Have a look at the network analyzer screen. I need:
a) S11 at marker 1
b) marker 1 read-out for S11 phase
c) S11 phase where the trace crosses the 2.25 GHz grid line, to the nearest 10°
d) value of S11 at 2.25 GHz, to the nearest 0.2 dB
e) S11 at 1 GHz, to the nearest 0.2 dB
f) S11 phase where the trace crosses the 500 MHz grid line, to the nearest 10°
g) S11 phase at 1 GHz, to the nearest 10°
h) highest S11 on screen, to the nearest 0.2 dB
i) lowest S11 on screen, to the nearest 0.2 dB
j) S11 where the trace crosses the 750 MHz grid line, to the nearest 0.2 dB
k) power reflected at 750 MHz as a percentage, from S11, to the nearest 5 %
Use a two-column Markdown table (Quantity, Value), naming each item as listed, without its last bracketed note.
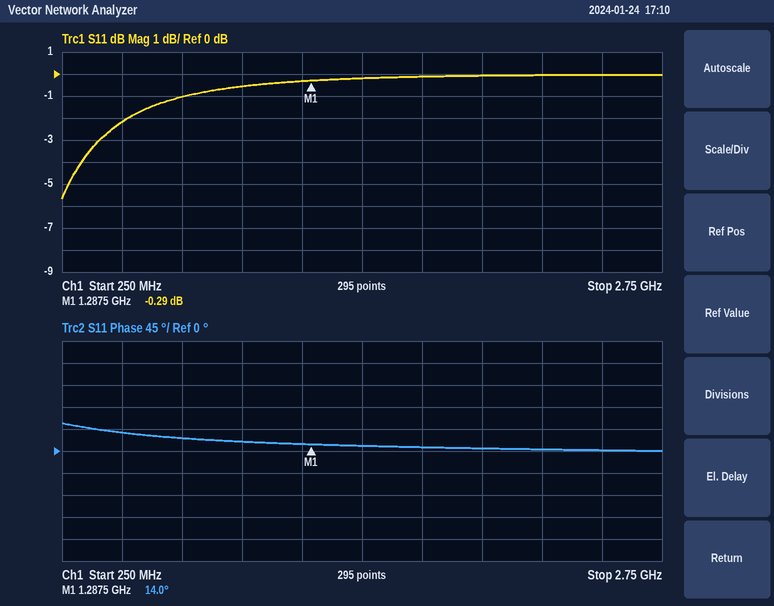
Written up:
| Quantity | Value |
|---|---|
| S11 at marker 1 | -0.29 dB |
| marker 1 read-out for S11 phase | 14.0° |
| S11 phase where the trace crosses the 2.25 GHz grid line, to the nearest 10° | 0° |
| value of S11 at 2.25 GHz, to the nearest 0.2 dB | 0.0 dB |
| S11 at 1 GHz, to the nearest 0.2 dB | -0.6 dB |
| S11 phase where the trace crosses the 500 MHz grid line, to the nearest 10° | 40° |
| S11 phase at 1 GHz, to the nearest 10° | 20° |
| highest S11 on screen, to the nearest 0.2 dB | 0.0 dB |
| lowest S11 on screen, to the nearest 0.2 dB | -5.6 dB |
| S11 where the trace crosses the 750 MHz grid line, to the nearest 0.2 dB | -1.0 dB |
| power reflected at 750 MHz as a percentage, from S11, to the nearest 5 % | 80 % |
